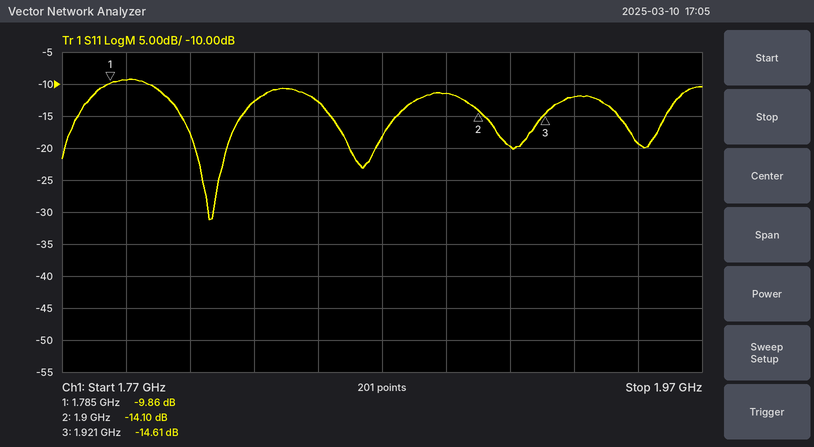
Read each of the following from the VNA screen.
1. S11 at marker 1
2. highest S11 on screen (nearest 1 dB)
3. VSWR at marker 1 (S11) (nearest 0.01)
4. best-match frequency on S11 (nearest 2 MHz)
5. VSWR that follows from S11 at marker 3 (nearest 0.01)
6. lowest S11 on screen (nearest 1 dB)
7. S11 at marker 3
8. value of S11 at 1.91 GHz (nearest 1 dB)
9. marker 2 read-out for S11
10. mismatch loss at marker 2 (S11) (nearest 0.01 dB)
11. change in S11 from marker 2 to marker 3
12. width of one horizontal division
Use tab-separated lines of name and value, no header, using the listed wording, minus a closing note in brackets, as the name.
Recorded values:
S11 at marker 1	-9.86 dB
highest S11 on screen	-9 dB
VSWR at marker 1 (S11)	1.95
best-match frequency on S11	1.816 GHz
VSWR that follows from S11 at marker 3	1.46
lowest S11 on screen	-31 dB
S11 at marker 3	-14.61 dB
value of S11 at 1.91 GHz	-20 dB
marker 2 read-out for S11	-14.10 dB
mismatch loss at marker 2 (S11)	0.17 dB
change in S11 from marker 2 to marker 3	-0.51 dB
width of one horizontal division	20 MHz
